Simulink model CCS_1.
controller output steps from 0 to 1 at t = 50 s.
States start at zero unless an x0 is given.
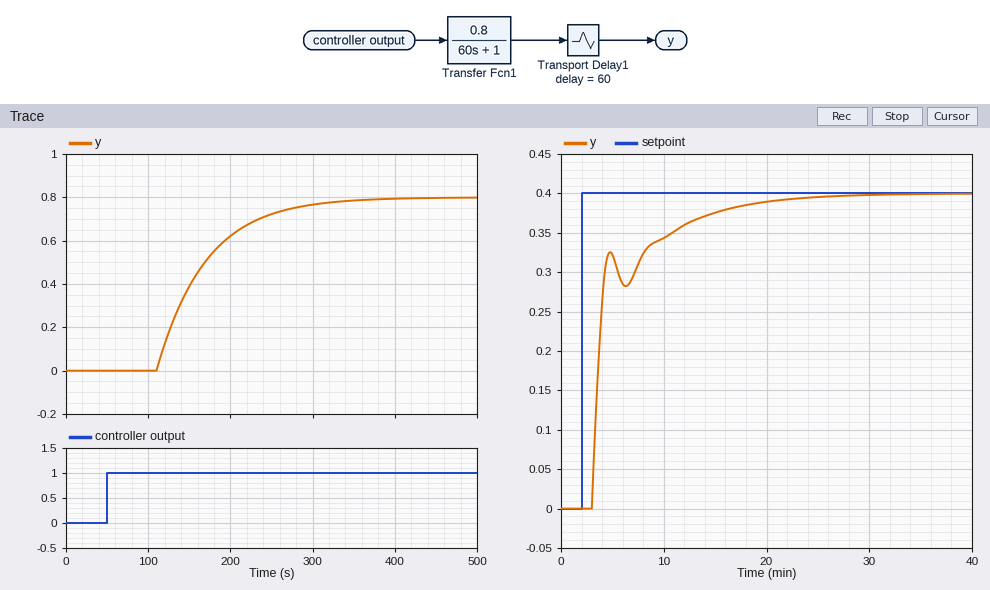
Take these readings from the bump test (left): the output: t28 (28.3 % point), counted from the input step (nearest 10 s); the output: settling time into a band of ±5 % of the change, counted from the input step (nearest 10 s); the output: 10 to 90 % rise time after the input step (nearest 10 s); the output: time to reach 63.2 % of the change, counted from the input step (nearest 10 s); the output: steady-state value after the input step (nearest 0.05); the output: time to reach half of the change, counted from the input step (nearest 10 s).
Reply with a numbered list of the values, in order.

1. 80 s
2. 240 s
3. 130 s
4. 120 s
5. 0.80
6. 100 s
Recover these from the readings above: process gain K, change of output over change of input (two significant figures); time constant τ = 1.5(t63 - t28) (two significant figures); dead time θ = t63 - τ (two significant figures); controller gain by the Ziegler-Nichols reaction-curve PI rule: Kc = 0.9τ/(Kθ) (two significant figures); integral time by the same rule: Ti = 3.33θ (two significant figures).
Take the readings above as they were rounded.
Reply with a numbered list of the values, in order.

1. 0.80
2. 60 s
3. 60 s
4. 1.1
5. 200 s
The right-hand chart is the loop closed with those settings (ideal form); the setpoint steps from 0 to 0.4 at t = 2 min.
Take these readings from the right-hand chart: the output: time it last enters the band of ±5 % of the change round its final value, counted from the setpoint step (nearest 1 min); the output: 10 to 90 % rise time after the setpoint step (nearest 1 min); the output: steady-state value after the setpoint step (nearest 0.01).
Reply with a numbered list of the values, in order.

1. 14 min
2. 9 min
3. 0.40
